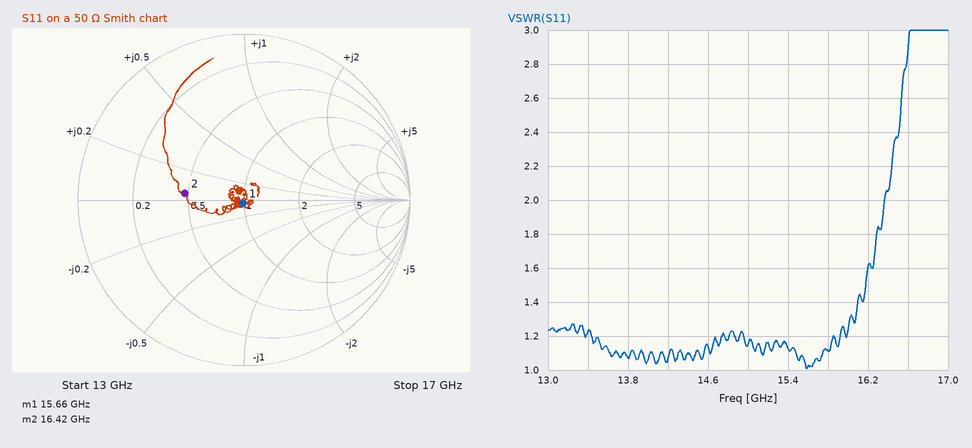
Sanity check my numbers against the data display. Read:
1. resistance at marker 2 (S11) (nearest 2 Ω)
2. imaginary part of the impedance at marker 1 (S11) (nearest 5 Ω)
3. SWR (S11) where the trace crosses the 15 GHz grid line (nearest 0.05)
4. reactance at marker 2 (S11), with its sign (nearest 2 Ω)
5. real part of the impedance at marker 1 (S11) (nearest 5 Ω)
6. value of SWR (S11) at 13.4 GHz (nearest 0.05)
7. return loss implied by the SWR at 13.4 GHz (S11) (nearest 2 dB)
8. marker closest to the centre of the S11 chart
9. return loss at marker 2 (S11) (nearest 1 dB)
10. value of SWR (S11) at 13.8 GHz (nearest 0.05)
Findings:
24 Ω
0 Ω
1.15
+2 Ω
50 Ω
1.25
20 dB
marker 1
9 dB
1.05
